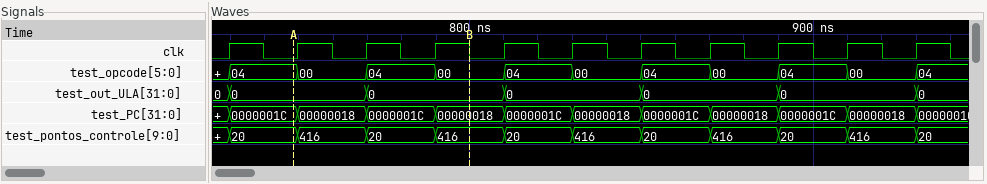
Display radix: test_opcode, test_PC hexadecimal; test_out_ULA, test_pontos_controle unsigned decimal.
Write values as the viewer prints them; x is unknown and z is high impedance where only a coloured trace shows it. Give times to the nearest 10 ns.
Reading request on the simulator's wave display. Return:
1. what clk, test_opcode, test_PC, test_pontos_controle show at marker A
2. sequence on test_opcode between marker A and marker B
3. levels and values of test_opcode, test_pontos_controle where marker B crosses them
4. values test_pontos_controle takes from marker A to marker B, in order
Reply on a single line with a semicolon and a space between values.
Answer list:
clk=0, test_opcode=04, test_PC=0000001C, test_pontos_controle=20; 04, 00, 04, 00; test_opcode=00, test_pontos_controle=416; 20, 416, 20, 416
